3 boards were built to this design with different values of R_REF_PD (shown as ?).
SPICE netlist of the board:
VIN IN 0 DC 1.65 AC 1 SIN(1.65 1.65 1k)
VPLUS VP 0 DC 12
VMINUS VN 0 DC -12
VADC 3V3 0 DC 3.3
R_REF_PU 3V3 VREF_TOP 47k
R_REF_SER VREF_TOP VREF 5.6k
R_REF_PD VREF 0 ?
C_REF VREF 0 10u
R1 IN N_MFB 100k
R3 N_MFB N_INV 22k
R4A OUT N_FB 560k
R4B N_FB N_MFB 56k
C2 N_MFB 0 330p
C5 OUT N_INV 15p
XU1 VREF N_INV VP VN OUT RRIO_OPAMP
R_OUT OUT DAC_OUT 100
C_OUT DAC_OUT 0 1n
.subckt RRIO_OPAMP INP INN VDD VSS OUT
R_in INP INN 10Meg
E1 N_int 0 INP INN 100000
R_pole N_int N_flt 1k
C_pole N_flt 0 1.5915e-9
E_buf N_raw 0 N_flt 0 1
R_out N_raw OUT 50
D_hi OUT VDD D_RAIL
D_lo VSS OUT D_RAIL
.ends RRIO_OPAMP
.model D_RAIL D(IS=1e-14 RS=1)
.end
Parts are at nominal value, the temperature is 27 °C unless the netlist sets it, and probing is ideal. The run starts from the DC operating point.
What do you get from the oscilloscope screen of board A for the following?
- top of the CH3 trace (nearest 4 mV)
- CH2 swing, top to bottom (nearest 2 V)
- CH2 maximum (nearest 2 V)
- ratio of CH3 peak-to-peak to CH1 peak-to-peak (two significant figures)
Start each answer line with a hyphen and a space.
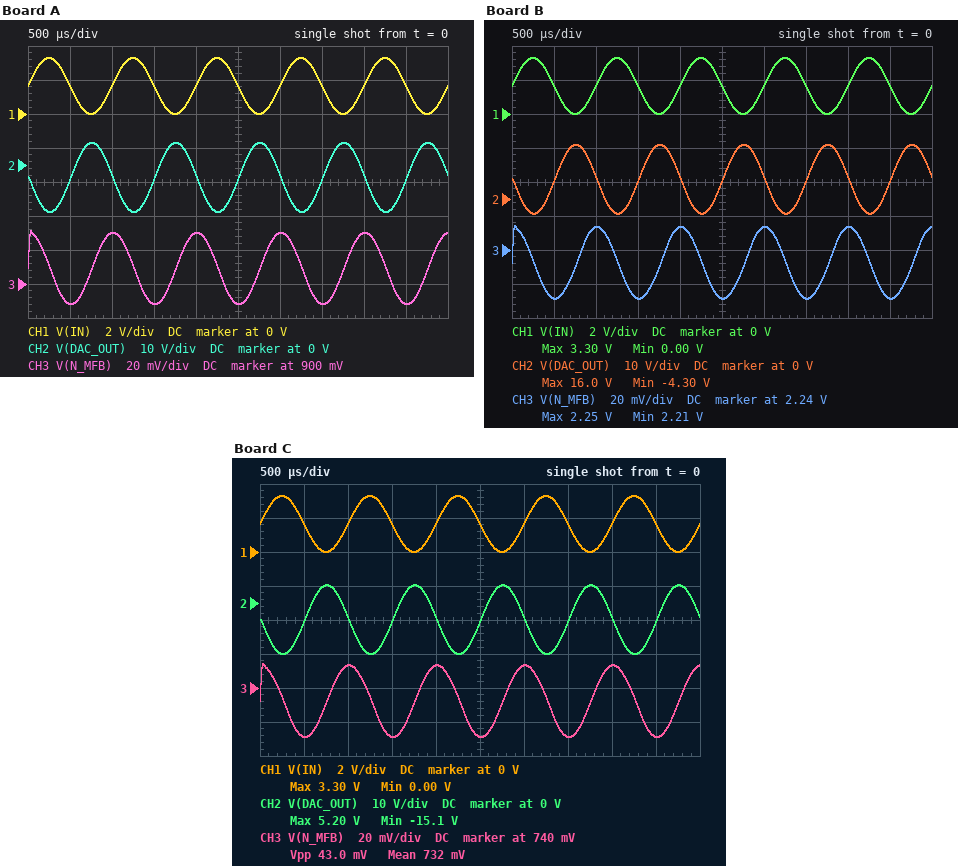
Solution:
- 932 mV
- 20 V
- 6 V
- 0.013
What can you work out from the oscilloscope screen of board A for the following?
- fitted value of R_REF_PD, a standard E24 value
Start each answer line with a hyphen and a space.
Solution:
- 20 kΩ
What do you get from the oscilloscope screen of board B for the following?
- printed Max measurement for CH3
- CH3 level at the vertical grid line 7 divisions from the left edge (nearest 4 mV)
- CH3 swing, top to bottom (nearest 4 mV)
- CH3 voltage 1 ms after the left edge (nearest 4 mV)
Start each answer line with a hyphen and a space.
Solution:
- 2.25 V
- 2.212 V
- 44 mV
- 2.252 V
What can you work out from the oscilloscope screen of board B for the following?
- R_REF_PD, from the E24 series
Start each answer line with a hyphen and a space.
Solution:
- 110 kΩ
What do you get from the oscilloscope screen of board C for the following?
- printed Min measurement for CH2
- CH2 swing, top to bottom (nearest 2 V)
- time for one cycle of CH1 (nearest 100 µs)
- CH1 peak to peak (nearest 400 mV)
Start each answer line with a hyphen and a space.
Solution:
- -15.1 V
- 20 V
- 1.0 ms
- 3.2 V
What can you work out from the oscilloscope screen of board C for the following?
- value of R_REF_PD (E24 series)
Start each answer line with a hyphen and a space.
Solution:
- 15 kΩ
